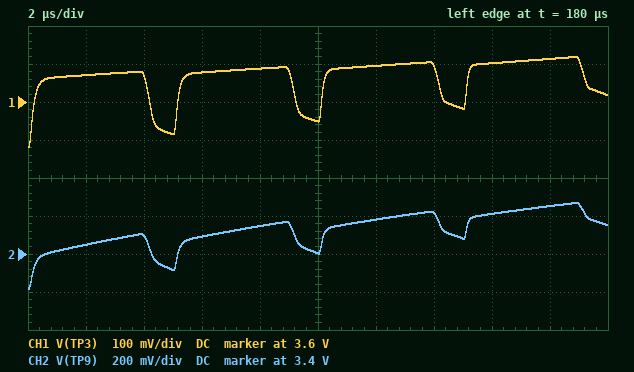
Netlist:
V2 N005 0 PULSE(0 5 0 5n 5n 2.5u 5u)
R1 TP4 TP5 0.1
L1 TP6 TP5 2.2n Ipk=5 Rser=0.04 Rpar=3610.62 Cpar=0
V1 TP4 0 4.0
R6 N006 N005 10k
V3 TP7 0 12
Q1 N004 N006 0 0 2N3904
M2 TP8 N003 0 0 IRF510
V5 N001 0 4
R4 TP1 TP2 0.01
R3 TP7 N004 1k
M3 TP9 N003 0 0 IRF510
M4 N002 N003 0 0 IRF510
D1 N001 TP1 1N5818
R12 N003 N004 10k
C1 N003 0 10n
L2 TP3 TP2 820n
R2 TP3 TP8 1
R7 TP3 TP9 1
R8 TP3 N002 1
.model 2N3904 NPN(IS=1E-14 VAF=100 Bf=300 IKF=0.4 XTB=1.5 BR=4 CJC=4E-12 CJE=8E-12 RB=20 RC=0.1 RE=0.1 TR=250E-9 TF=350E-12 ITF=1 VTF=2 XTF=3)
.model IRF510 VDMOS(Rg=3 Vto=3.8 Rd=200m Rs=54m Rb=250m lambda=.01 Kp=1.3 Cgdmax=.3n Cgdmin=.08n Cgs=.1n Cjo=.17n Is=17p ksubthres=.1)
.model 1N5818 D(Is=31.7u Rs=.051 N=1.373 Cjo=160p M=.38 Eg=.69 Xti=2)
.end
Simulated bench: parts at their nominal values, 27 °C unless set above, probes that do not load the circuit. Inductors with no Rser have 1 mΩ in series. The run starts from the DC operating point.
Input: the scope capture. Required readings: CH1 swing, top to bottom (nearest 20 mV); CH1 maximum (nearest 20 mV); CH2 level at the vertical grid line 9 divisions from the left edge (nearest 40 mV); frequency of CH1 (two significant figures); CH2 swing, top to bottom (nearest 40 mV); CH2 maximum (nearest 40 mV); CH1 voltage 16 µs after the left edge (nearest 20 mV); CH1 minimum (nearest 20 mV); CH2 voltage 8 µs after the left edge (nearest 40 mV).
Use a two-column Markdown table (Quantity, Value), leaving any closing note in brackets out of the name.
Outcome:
| Quantity | Value |
|---|---|
| CH1 swing, top to bottom | 240 mV |
| CH1 maximum | 3.72 V |
| CH2 level at the vertical grid line 9 divisions from the left edge | 3.64 V |
| frequency of CH1 | 200 kHz |
| CH2 swing, top to bottom | 440 mV |
| CH2 maximum | 3.68 V |
| CH1 voltage 16 µs after the left edge | 3.70 V |
| CH1 minimum | 3.48 V |
| CH2 voltage 8 µs after the left edge | 3.56 V |
